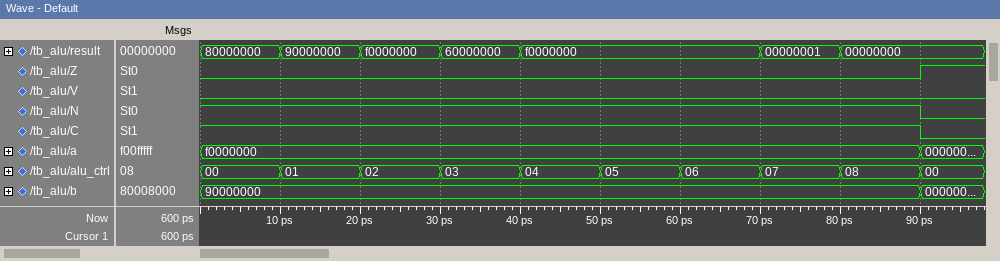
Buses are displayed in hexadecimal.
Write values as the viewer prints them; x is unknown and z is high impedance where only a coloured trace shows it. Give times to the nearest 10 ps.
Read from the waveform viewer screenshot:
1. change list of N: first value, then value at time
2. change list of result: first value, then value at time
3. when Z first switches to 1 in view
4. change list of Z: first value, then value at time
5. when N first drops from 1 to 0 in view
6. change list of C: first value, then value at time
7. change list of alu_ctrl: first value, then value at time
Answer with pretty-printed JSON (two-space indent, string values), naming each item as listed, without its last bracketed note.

{
  "change list of N: first value, then value at time": "1, 0 at 90 ps",
  "change list of result: first value, then value at time": "80000000, 90000000 at 10 ps, f0000000 at 20 ps, 60000000 at 30 ps, f0000000 at 40 ps, 00000001 at 70 ps, 00000000 at 80 ps",
  "when Z first switches to 1 in view": "90 ps",
  "change list of Z: first value, then value at time": "0, 1 at 90 ps",
  "when N first drops from 1 to 0 in view": "90 ps",
  "change list of C: first value, then value at time": "1, 0 at 90 ps",
  "change list of alu_ctrl: first value, then value at time": "00, 01 at 10 ps, 02 at 20 ps, 03 at 30 ps, 04 at 40 ps, 05 at 50 ps, 06 at 60 ps, 07 at 70 ps, 08 at 80 ps, 00 at 90 ps"
}
